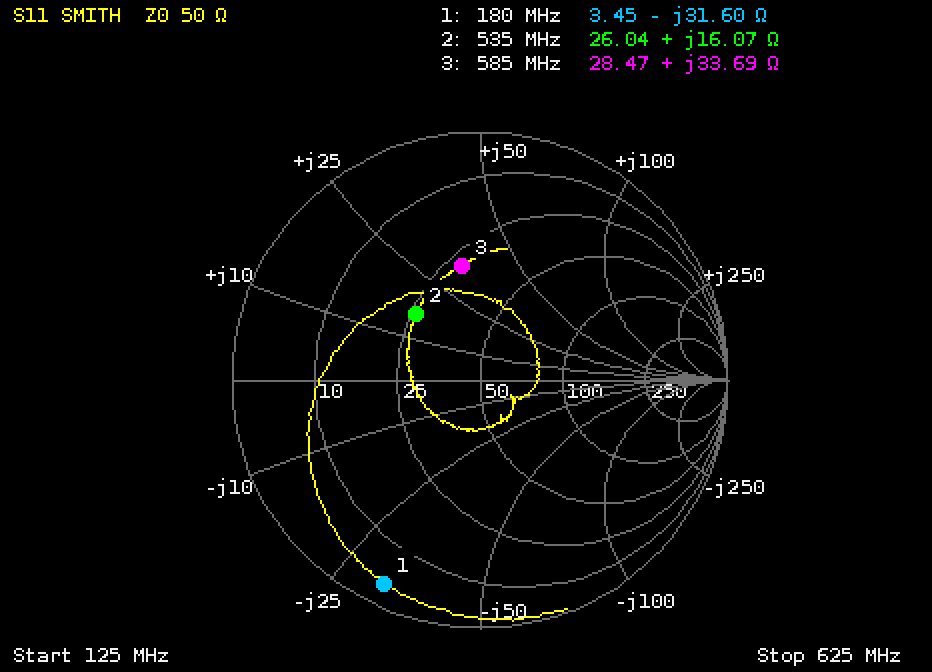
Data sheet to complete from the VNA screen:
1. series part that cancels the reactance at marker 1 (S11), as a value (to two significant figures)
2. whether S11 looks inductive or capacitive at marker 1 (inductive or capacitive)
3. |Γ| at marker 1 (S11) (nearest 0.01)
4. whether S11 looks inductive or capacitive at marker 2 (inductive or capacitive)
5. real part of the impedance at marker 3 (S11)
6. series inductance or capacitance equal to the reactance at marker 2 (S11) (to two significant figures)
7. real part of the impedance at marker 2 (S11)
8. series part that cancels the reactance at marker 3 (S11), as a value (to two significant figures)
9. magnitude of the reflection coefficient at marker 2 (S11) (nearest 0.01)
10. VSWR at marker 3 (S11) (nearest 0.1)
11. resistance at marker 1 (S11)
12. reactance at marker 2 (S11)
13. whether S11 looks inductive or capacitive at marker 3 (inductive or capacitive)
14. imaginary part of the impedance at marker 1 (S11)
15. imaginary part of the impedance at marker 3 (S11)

28 nH
capacitive
0.91
inductive
28.47 Ω
4.8 nH
26.04 Ω
8.1 pF
0.37
2.8
3.45 Ω
+16.07 Ω
inductive
-31.60 Ω
+33.69 Ω
